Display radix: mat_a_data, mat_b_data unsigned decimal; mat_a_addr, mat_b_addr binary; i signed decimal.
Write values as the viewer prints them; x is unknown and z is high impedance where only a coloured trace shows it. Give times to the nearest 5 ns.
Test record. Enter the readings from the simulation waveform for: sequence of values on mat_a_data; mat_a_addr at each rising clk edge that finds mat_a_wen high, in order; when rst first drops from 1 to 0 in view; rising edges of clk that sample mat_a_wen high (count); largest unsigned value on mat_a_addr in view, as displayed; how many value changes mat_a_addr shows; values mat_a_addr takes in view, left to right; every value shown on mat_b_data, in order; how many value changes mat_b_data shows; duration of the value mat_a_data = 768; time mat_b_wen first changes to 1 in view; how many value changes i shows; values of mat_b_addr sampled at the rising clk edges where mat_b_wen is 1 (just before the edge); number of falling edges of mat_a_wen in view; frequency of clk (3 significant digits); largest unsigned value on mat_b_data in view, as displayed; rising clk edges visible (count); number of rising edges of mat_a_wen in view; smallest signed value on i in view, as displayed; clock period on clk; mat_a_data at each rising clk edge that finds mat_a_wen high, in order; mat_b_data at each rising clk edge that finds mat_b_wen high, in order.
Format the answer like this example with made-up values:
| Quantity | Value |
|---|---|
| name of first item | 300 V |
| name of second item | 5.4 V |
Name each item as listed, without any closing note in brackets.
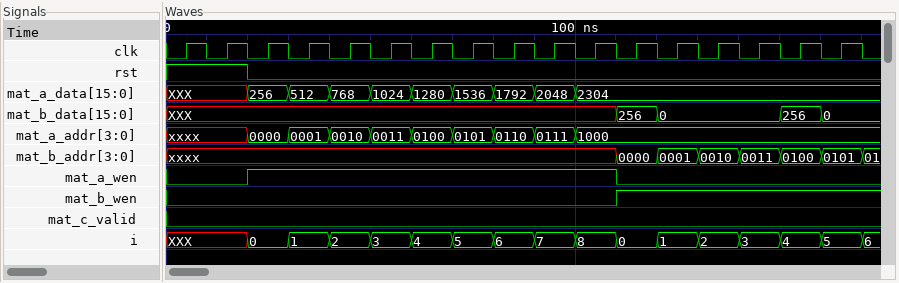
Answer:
| Quantity | Value |
|---|---|
| sequence of values on mat_a_data | XXX, 256, 512, 768, 1024, 1280, 1536, 1792, 2048, 2304 |
| mat_a_addr at each rising clk edge that finds mat_a_wen high, in order | 0000, 0001, 0010, 0011, 0100, 0101, 0110, 0111, 1000 |
| when rst first drops from 1 to 0 in view | 20 ns |
| rising edges of clk that sample mat_a_wen high | 9 |
| largest unsigned value on mat_a_addr in view, as displayed | 1000 |
| how many value changes mat_a_addr shows | 9 |
| values mat_a_addr takes in view, left to right | xxxx, 0000, 0001, 0010, 0011, 0100, 0101, 0110, 0111, 1000 |
| every value shown on mat_b_data, in order | XXX, 256, 0, 256, 0 |
| how many value changes mat_b_data shows | 4 |
| duration of the value mat_a_data = 768 | 10 ns |
| time mat_b_wen first changes to 1 in view | 110 ns |
| how many value changes i shows | 16 |
| values of mat_b_addr sampled at the rising clk edges where mat_b_wen is 1 | 0000, 0001, 0010, 0011, 0100, 0101 |
| number of falling edges of mat_a_wen in view | 1 |
| frequency of clk | 100 MHz |
| largest unsigned value on mat_b_data in view, as displayed | 256 |
| rising clk edges visible | 17 |
| number of rising edges of mat_a_wen in view | 1 |
| smallest signed value on i in view, as displayed | 0 |
| clock period on clk | 10 ns |
| mat_a_data at each rising clk edge that finds mat_a_wen high, in order | 256, 512, 768, 1024, 1280, 1536, 1792, 2048, 2304 |
| mat_b_data at each rising clk edge that finds mat_b_wen high, in order | 256, 0, 0, 0, 256, 0 |
